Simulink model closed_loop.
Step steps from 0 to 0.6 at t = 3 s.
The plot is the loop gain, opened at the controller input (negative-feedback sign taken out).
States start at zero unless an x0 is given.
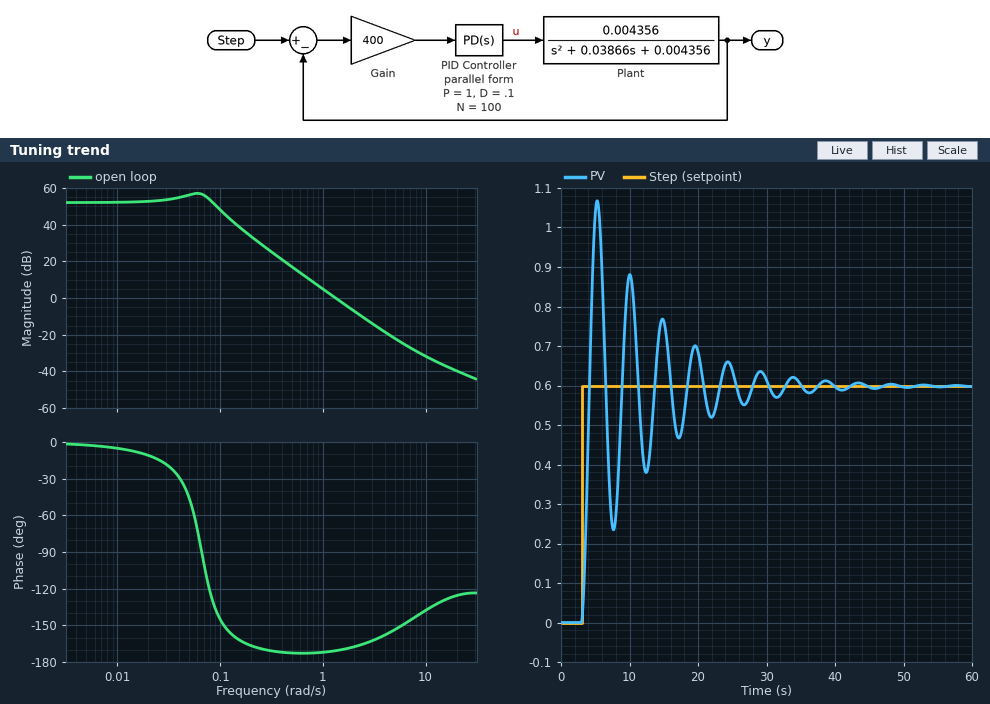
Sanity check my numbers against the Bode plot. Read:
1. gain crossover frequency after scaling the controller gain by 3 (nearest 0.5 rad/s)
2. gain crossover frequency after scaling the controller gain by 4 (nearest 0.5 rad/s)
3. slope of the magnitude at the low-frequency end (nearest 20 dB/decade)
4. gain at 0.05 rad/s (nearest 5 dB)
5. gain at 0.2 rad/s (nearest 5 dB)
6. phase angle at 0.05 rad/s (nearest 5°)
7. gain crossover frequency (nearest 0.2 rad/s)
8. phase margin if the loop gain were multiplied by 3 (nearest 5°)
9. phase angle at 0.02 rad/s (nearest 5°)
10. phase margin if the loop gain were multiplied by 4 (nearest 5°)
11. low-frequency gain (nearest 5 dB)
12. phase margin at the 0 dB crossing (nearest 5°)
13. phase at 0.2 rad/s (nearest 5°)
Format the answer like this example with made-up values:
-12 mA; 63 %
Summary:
2.5 rad/s; 2.5 rad/s; 0 dB/decade; 55 dB; 35 dB; -45°; 1.4 rad/s; 15°; -10°; 15°; 50 dB; 10°; -165°
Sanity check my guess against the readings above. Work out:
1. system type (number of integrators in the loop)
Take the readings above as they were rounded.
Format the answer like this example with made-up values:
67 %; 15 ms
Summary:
0
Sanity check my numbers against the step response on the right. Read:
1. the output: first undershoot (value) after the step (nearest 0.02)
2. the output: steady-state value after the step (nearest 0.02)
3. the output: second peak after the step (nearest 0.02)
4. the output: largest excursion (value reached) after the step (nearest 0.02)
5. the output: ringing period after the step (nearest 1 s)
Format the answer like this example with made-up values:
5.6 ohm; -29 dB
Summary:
0.24; 0.60; 0.88; 1.06; 5 s
